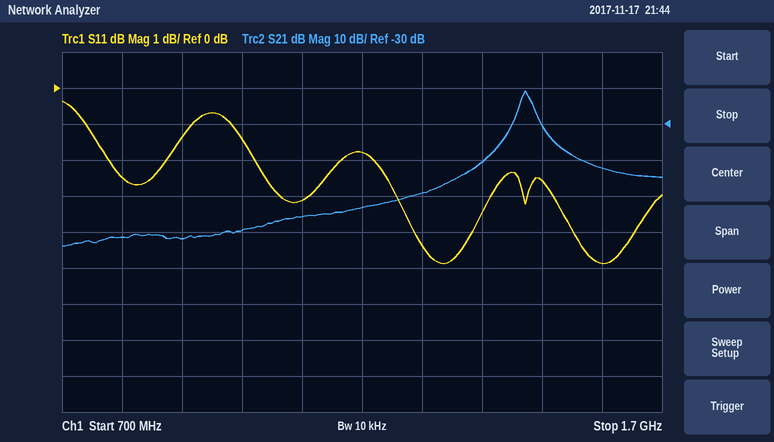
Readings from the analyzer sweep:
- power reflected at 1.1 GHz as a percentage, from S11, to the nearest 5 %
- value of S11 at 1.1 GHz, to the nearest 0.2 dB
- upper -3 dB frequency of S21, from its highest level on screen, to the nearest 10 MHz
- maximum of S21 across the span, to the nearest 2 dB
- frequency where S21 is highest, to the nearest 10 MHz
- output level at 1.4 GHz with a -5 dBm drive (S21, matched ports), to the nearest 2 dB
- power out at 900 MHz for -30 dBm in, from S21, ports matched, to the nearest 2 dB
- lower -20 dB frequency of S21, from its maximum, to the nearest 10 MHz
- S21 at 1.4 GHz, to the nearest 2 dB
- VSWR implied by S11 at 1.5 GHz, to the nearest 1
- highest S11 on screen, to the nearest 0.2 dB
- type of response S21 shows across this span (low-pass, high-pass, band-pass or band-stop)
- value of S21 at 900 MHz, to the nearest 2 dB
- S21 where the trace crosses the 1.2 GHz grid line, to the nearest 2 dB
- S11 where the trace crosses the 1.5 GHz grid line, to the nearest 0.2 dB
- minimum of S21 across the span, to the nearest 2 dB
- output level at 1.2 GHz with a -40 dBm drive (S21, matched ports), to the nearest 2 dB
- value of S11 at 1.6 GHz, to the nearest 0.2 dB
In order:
50 %
-3.2 dB
1.48 GHz
-20 dB
1.47 GHz
-46 dBm
-92 dBm
1.40 GHz
-40 dB
7
-0.4 dB
band-pass
-62 dB
-54 dB
-2.6 dB
-64 dB
-94 dBm
-4.8 dB
